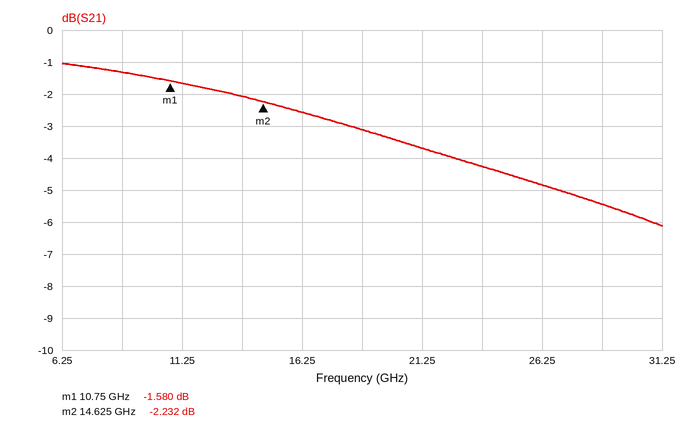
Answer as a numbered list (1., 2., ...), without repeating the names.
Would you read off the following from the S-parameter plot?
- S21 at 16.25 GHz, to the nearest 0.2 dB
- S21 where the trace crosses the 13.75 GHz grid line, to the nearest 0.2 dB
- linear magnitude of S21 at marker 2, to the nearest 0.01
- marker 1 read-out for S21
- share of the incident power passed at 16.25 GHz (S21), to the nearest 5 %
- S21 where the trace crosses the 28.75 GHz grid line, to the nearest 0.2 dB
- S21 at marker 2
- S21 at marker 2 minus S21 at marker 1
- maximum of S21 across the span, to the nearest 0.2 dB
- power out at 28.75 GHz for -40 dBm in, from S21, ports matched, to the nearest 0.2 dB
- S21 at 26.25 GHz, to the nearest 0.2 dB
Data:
1. -2.6 dB
2. -2.0 dB
3. 0.77
4. -1.580 dB
5. 55 %
6. -5.4 dB
7. -2.232 dB
8. -0.652 dB
9. -1.0 dB
10. -45.4 dBm
11. -4.8 dB
